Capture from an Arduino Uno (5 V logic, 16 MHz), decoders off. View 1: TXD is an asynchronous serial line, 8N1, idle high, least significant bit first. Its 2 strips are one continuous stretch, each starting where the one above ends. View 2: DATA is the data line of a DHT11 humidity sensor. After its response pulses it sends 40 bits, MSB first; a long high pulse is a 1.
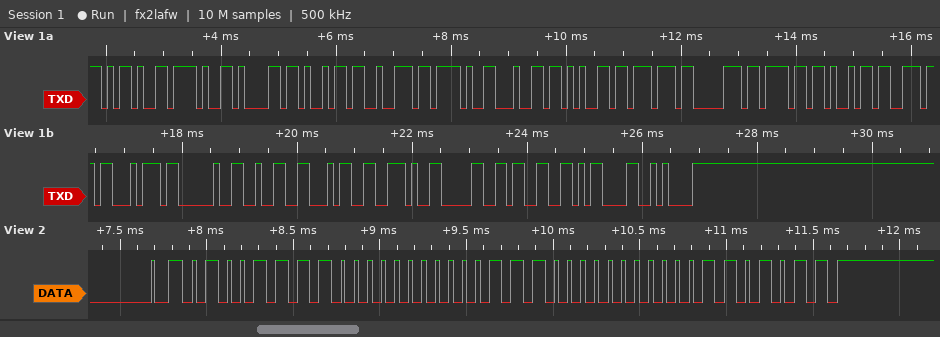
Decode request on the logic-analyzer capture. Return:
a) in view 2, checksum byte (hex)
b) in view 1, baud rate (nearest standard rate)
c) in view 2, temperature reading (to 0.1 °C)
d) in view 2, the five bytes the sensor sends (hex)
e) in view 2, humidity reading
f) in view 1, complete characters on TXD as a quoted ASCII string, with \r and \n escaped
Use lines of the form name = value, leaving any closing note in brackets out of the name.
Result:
in view 2, checksum byte = 0x6B
in view 1, baud rate = 9600 baud
in view 2, temperature reading = 28.0 °C
in view 2, the five bytes the sensor sends = 4F 00 1C 00 6B
in view 2, humidity reading = 79 %
in view 1, complete characters on TXD as a quoted ASCII string, with \r and \n escaped = "-/air/dewpoint 24.03\r\n"
